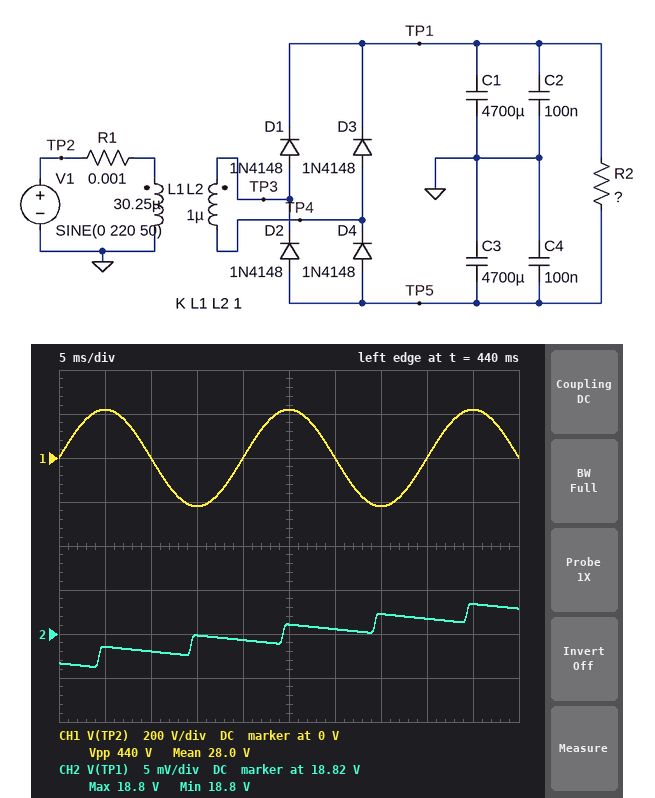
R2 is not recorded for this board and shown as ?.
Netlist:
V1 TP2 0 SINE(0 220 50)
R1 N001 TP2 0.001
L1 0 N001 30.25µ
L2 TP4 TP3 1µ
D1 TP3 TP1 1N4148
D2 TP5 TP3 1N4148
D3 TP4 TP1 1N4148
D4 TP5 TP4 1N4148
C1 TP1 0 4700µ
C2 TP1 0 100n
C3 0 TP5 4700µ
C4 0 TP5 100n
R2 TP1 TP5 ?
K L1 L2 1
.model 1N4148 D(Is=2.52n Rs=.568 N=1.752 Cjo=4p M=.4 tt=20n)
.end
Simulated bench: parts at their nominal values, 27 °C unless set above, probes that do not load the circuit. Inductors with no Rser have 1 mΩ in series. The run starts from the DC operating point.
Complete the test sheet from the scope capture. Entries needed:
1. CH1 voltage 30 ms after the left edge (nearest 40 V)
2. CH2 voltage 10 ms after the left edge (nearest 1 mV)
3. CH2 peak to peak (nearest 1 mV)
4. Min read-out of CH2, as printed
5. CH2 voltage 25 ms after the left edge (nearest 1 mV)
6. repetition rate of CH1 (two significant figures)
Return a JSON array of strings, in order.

["0 V", "18.823 V", "7 mV", "18.8 V", "18.826 V", "50 Hz"]
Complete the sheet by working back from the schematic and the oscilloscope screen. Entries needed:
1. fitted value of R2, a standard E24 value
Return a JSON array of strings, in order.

["75 kΩ"]
